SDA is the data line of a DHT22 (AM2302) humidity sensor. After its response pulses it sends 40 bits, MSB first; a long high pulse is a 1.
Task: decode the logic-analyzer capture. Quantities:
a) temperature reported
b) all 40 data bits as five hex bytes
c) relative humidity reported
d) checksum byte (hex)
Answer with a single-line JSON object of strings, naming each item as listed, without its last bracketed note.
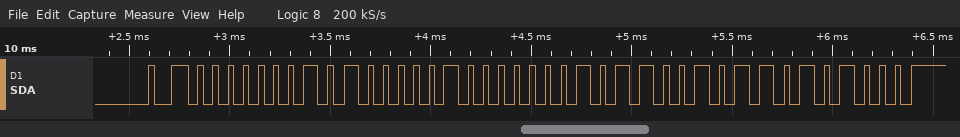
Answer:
{"temperature reported": "35.7 °C", "all 40 data bits as five hex bytes": "01 41 01 65 A8", "relative humidity reported": "32.1 %", "checksum byte": "0xA8"}
